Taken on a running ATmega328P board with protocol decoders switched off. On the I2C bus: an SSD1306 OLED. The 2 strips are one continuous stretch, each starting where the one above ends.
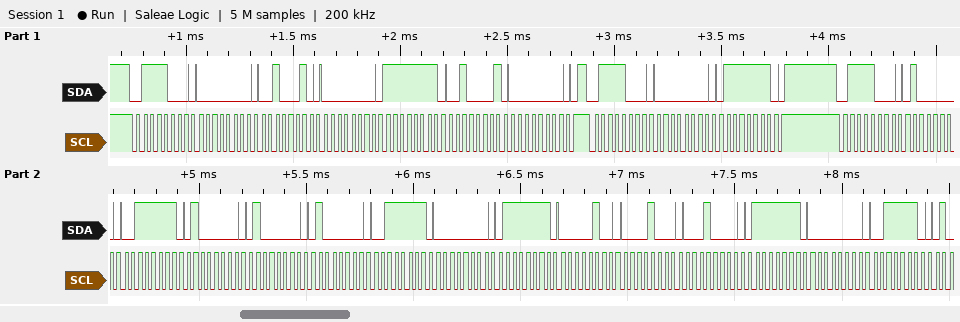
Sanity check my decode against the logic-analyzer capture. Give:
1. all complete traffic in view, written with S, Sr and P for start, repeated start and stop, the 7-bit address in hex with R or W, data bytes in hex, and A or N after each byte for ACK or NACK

S 3CW A 00 A 22 A 00 A FF A 21 A 00 A P S 3CW A 00 A 7F A P S 3CW A 40 A 3F A 40 A 40 A 40 A 3F A 00 A 7F A 04 A 08 A 10 A 7F A 00 A 3E A
